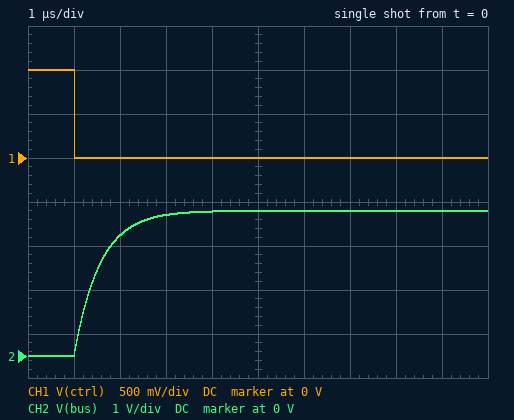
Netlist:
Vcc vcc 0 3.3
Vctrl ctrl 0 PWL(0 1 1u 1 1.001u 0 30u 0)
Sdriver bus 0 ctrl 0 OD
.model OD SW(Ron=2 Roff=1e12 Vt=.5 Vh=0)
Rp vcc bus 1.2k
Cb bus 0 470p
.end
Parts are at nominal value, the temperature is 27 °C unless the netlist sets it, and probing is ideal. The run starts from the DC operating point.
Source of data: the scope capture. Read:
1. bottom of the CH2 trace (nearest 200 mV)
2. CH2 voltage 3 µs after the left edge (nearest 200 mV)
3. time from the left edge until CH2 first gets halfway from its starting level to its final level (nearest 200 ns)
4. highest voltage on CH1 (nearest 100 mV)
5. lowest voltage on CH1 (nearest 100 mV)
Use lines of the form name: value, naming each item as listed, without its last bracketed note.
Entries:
bottom of the CH2 trace: 0 V
CH2 voltage 3 µs after the left edge: 3.2 V
time from the left edge until CH2 first gets halfway from its starting level to its final level: 1.4 µs
highest voltage on CH1: 1.0 V
lowest voltage on CH1: 0 V
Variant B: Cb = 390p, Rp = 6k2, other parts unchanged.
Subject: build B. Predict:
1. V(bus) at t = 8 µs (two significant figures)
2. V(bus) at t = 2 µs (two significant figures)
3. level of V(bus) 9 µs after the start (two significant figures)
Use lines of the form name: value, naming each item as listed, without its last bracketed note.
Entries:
V(bus) at t = 8 µs: 3.1 V
V(bus) at t = 2 µs: 1.1 V
level of V(bus) 9 µs after the start: 3.2 V
